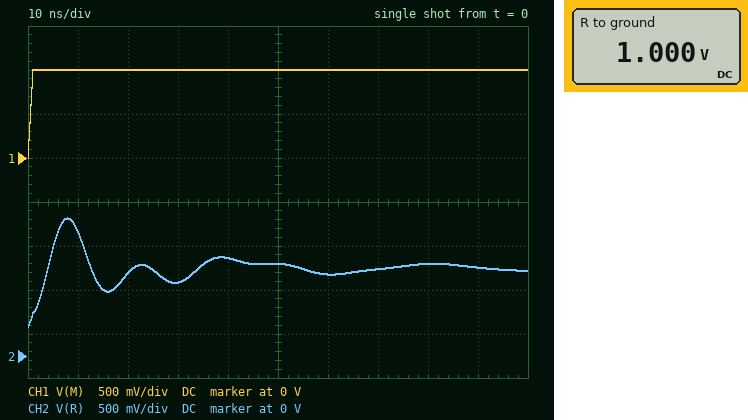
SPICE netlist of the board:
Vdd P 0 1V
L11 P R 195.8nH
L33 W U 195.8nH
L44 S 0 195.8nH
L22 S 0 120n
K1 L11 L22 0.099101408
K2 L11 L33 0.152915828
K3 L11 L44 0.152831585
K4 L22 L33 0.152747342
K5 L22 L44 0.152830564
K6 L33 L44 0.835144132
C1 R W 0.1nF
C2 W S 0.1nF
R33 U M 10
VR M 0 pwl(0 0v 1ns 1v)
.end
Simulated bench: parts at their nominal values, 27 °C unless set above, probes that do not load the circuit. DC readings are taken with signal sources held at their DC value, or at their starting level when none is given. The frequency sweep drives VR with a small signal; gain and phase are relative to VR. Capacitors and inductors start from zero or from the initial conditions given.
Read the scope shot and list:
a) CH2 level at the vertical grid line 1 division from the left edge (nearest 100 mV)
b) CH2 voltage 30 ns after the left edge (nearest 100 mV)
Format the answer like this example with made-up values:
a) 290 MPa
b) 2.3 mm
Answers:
a) 1.4 V
b) 800 mV
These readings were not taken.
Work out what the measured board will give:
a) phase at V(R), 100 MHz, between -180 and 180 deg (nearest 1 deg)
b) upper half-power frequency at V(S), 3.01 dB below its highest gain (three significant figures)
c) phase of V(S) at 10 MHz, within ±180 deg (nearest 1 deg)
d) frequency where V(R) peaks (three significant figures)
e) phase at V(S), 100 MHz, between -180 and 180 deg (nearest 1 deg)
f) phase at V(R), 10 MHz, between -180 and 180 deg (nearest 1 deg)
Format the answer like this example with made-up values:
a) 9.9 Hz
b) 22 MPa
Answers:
a) -155 deg
b) 78.1 MHz
c) -8 deg
d) 26.9 MHz
e) 25 deg
f) 172 deg
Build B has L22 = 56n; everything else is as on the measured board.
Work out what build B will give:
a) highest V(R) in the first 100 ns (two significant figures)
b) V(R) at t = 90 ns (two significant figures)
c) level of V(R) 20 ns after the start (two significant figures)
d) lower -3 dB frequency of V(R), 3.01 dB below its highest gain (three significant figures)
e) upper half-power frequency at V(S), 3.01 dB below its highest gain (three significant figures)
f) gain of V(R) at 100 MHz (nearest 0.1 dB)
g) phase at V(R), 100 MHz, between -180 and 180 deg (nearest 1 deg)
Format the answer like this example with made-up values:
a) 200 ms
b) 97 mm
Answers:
a) 1.7 V
b) 980 mV
c) 1.0 V
d) 25.5 MHz
e) 80.6 MHz
f) -5.9 dB
g) -154 deg
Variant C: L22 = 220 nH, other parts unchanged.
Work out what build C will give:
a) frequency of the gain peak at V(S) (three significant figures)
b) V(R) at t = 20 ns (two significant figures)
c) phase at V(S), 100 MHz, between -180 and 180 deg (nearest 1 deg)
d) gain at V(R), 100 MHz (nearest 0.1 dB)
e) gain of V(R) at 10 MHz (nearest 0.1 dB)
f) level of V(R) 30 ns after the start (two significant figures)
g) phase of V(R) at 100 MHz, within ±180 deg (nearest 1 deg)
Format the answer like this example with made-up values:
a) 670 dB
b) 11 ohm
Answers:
a) 25.9 MHz
b) 910 mV
c) 24 deg
d) -17.3 dB
e) -19.6 dB
f) 850 mV
g) -156 deg
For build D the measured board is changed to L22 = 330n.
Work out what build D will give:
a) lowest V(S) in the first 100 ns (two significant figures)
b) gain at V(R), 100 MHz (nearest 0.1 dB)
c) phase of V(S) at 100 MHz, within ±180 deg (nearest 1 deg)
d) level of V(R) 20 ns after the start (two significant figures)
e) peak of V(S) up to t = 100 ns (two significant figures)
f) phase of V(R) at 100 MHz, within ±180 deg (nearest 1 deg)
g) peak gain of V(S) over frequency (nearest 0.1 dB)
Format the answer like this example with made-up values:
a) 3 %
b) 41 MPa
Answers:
a) -490 mV
b) -23.4 dB
c) 23 deg
d) 910 mV
e) 580 mV
f) -157 deg
g) 6.4 dB
